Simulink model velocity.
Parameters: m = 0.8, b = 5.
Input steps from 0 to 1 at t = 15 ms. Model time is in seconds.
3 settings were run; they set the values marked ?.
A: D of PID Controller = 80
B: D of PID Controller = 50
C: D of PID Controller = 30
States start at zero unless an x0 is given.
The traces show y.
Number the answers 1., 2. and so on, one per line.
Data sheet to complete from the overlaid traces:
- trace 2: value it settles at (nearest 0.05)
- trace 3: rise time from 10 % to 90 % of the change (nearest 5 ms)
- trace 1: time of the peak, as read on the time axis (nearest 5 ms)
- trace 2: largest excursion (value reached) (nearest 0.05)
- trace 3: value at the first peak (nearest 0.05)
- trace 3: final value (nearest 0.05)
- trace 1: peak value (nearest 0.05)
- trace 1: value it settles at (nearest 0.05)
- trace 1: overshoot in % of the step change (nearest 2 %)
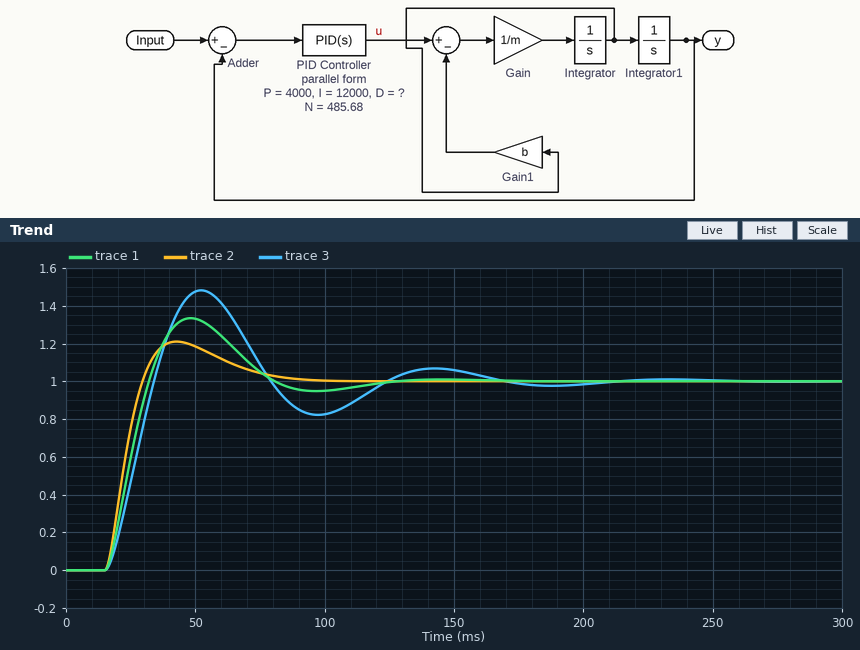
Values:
1. 1.00
2. 15 ms
3. 50 ms
4. 1.20
5. 1.50
6. 1.00
7. 1.35
8. 1.00
9. 34 %
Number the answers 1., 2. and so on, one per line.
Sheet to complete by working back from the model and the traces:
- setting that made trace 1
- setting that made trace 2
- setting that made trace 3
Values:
1. B
2. A
3. C
